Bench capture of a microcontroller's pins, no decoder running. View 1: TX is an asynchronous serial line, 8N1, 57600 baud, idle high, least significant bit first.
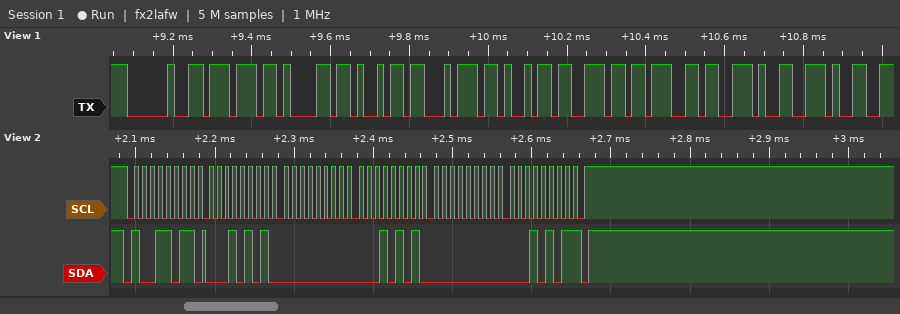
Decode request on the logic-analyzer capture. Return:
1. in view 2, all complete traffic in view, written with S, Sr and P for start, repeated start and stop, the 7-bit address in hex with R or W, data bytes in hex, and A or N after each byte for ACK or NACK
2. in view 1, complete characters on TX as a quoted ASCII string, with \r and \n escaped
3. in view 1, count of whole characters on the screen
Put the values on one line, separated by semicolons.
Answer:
S 4DR A 15 A 00 A 15 A 00 A 15 N P; " waiting.."; 10
